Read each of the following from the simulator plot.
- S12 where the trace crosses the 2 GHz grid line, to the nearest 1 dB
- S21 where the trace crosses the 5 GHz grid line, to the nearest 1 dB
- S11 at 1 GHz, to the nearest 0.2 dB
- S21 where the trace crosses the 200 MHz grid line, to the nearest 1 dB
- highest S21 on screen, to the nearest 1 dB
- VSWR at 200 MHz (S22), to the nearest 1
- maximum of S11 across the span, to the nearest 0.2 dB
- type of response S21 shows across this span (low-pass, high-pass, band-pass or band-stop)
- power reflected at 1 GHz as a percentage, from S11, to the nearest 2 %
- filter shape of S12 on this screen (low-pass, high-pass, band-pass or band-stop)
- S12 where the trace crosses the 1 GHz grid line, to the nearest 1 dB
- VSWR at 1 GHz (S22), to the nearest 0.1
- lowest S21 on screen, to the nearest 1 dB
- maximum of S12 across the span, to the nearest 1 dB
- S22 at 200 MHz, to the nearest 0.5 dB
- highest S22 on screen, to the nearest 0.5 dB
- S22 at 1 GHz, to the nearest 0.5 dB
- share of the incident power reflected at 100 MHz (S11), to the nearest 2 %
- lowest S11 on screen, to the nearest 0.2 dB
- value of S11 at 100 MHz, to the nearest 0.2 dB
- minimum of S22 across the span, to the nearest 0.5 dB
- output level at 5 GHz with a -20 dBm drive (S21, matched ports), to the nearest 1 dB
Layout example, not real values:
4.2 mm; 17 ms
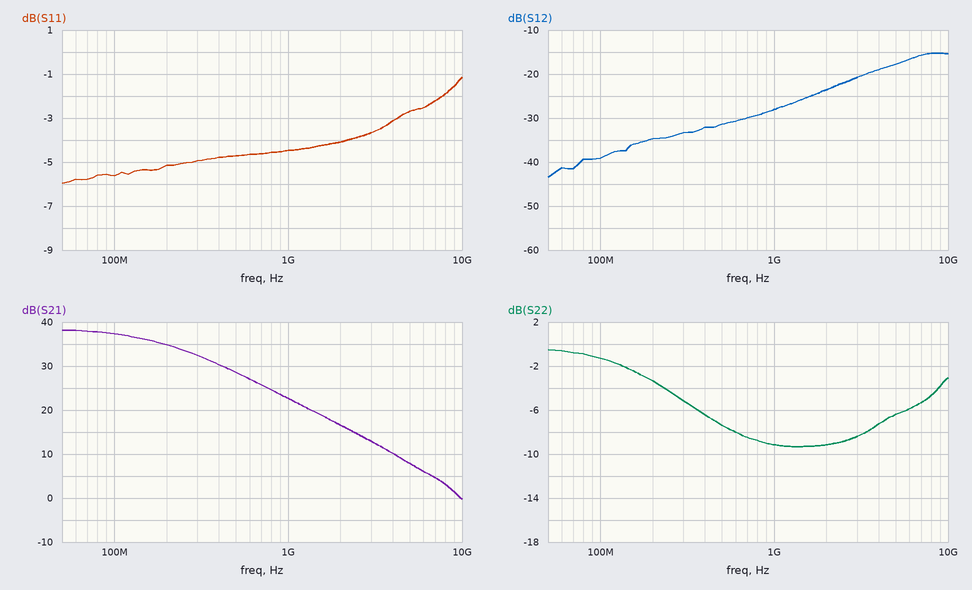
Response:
-24 dB; 8 dB; -4.4 dB; 35 dB; 38 dB; 5; -1.2 dB; low-pass; 36 %; high-pass; -28 dB; 2.1; 0 dB; -15 dB; -3.5 dB; -0.5 dB; -9.0 dB; 28 %; -6.0 dB; -5.6 dB; -9.5 dB; -12 dBm
